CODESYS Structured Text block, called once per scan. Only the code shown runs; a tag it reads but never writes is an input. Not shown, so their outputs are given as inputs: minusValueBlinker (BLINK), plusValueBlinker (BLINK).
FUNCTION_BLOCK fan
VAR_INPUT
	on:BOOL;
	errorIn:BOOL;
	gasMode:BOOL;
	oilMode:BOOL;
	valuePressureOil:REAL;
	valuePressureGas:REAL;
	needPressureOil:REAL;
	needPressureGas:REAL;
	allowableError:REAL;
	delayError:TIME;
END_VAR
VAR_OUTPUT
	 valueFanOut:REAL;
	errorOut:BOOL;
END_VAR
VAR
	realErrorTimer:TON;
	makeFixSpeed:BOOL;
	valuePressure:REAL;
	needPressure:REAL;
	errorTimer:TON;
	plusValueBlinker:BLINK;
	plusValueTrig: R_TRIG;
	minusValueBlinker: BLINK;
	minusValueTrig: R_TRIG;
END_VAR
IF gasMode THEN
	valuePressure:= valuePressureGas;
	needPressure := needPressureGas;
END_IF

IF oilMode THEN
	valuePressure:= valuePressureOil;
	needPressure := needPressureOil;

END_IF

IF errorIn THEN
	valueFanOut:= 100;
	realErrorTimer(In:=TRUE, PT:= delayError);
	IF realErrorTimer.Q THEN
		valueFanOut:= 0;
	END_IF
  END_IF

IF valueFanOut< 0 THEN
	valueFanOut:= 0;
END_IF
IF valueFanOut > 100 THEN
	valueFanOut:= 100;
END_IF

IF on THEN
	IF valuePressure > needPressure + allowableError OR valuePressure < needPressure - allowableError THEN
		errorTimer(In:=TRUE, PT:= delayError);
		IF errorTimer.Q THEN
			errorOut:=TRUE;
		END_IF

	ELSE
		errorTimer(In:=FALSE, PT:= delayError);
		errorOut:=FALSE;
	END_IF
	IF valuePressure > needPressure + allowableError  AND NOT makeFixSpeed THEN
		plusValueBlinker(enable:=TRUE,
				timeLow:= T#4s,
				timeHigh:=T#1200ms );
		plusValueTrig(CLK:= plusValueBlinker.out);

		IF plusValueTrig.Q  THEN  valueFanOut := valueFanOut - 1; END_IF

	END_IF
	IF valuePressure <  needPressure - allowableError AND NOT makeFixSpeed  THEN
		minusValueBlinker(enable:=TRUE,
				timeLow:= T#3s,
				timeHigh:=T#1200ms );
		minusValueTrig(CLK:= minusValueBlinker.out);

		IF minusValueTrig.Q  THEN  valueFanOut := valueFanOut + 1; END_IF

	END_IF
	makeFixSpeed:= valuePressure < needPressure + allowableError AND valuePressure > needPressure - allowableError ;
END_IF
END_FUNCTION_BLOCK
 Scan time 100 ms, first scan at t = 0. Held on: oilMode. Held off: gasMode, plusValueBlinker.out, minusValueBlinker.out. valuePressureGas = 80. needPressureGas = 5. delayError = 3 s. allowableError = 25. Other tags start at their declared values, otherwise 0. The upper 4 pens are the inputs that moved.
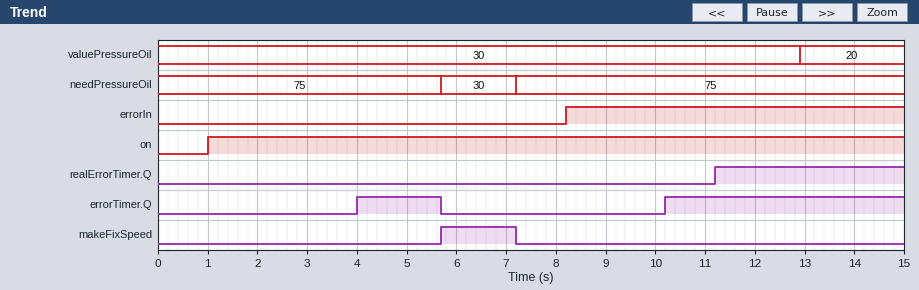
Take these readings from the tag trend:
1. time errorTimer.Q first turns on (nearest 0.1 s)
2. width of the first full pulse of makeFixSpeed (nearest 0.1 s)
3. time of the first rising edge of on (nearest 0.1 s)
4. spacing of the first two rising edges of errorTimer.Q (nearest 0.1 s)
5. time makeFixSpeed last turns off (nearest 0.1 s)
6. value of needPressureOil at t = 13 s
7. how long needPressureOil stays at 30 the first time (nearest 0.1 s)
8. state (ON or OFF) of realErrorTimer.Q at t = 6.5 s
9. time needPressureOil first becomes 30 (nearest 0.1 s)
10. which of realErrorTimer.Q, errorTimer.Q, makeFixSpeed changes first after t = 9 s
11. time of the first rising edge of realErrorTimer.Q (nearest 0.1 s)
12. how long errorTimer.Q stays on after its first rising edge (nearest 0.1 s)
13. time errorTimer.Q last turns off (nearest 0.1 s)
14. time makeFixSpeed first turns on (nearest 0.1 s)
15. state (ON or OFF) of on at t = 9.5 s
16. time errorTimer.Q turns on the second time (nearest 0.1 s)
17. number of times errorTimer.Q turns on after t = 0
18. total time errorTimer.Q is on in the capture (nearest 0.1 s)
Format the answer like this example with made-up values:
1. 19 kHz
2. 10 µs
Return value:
1. 4.0 s
2. 1.5 s
3. 1.0 s
4. 6.2 s
5. 7.2 s
6. 75
7. 1.5 s
8. OFF
9. 5.7 s
10. errorTimer.Q
11. 11.2 s
12. 1.7 s
13. 5.7 s
14. 5.7 s
15. ON
16. 10.2 s
17. 2
18. 6.5 s
